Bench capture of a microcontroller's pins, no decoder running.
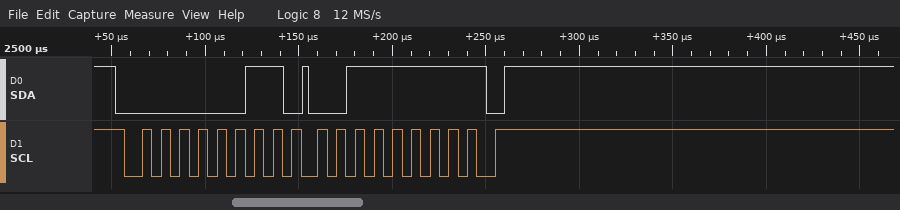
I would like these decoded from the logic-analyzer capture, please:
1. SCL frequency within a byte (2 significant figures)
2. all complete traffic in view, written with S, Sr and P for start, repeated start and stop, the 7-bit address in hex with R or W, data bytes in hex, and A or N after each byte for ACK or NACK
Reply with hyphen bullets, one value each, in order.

- 100 kHz
- S 01R A 3F N P
